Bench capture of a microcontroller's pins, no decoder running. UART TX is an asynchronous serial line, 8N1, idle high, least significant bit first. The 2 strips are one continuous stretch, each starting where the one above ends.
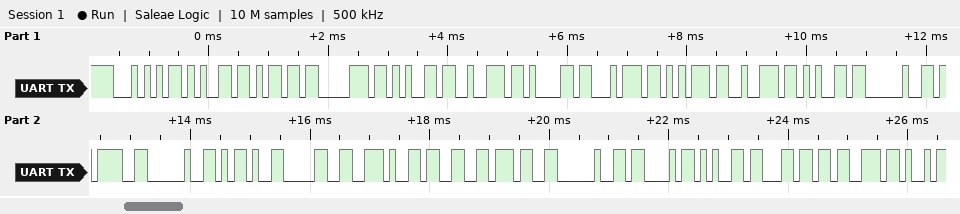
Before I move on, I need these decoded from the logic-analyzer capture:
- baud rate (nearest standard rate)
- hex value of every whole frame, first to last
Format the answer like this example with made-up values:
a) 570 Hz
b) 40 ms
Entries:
a) 9600 baud
b) 54 65 6D 70 65 72 61 74 75 72 65 20 3D 20 2D 30 2E 33 37 20 43 65 6C 73
